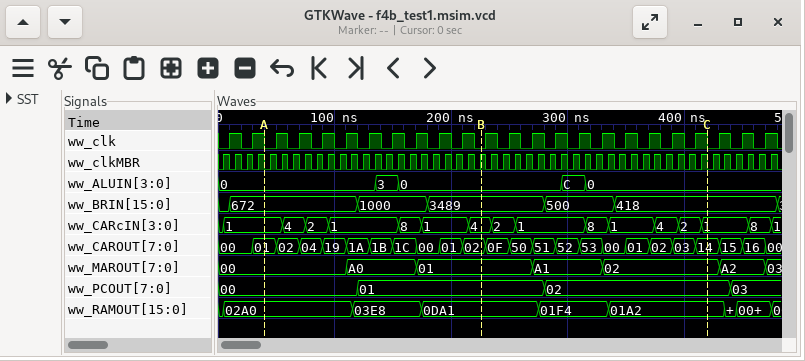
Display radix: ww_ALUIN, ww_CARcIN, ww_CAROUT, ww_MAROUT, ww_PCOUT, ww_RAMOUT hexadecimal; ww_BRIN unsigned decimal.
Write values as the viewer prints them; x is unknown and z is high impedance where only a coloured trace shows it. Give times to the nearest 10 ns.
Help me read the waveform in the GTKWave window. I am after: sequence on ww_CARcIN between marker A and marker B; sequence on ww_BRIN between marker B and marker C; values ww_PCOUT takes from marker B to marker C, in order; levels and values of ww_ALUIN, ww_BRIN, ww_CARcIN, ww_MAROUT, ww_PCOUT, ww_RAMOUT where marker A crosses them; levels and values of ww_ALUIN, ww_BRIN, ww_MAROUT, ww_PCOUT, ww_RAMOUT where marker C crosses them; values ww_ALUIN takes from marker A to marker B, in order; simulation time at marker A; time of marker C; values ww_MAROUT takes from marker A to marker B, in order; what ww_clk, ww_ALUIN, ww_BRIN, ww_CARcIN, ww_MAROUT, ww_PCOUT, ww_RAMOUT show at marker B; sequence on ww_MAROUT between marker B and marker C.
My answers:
1, 4, 2, 1, 8, 1, 4
3489, 500, 418
01, 02
ww_ALUIN=0, ww_BRIN=672, ww_CARcIN=1, ww_MAROUT=00, ww_PCOUT=00, ww_RAMOUT=02A0
ww_ALUIN=0, ww_BRIN=418, ww_MAROUT=02, ww_PCOUT=02, ww_RAMOUT=01A2
0, 3, 0
40 ns
420 ns
00, A0, 01
ww_clk=0, ww_ALUIN=0, ww_BRIN=3489, ww_CARcIN=4, ww_MAROUT=01, ww_PCOUT=01, ww_RAMOUT=0DA1
01, A1, 02
